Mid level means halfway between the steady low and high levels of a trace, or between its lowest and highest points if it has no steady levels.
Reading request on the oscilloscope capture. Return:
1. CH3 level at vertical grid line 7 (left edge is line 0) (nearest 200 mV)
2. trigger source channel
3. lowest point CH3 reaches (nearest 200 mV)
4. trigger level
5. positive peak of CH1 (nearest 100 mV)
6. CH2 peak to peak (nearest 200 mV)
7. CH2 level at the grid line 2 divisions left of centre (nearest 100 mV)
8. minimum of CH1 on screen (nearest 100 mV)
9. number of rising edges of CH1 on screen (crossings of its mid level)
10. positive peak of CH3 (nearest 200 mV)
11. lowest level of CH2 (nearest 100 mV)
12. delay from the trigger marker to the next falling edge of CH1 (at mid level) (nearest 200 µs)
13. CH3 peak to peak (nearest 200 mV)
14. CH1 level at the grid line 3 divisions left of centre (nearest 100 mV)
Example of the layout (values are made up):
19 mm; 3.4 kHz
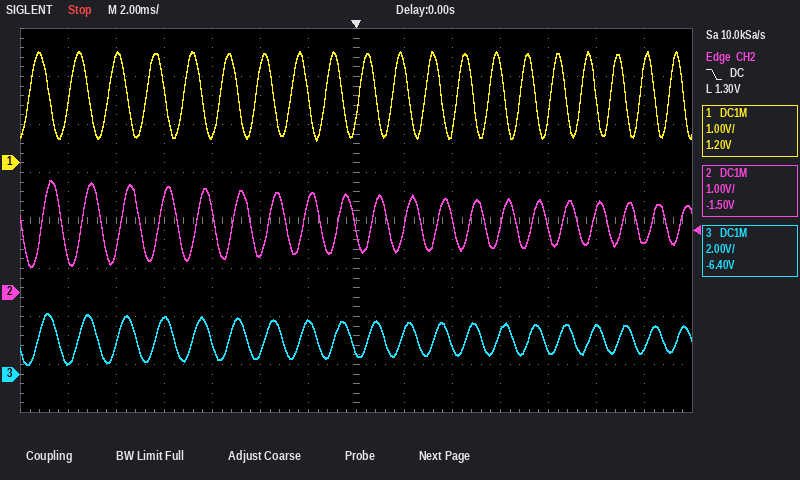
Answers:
1.0 V; CH2; 400 mV; 1.30 V; 2.3 V; 1.8 V; 800 mV; 500 mV; 20; 2.6 V; 500 mV; 800 µs; 2.2 V; 600 mV
